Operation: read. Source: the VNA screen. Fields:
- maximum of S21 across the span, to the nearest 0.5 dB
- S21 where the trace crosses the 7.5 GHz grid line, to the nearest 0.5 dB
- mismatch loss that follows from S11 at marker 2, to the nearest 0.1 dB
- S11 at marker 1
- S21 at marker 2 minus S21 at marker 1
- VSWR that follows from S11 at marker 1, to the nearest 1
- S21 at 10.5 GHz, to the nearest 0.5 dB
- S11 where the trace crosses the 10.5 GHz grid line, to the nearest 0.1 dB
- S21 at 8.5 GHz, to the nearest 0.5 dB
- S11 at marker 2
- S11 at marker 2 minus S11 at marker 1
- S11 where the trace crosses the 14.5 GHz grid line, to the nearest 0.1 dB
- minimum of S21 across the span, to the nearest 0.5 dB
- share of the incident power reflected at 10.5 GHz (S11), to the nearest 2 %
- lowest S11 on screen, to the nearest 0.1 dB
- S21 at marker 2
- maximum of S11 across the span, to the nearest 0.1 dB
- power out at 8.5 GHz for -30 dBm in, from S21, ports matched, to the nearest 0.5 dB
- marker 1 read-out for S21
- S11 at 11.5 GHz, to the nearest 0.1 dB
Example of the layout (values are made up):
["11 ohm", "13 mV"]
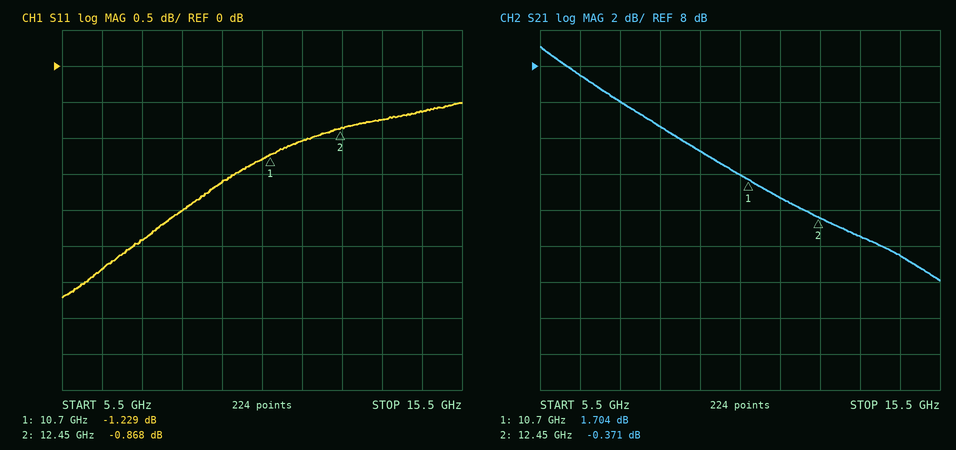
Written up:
["9.0 dB", "6.0 dB", "7.4 dB", "-1.229 dB", "-2.075 dB", "14", "2.0 dB", "-1.3 dB", "4.5 dB", "-0.868 dB", "0.361 dB", "-0.6 dB", "-4.0 dB", "74 %", "-3.2 dB", "-0.371 dB", "-0.5 dB", "-25.5 dBm", "1.704 dB", "-1.0 dB"]
